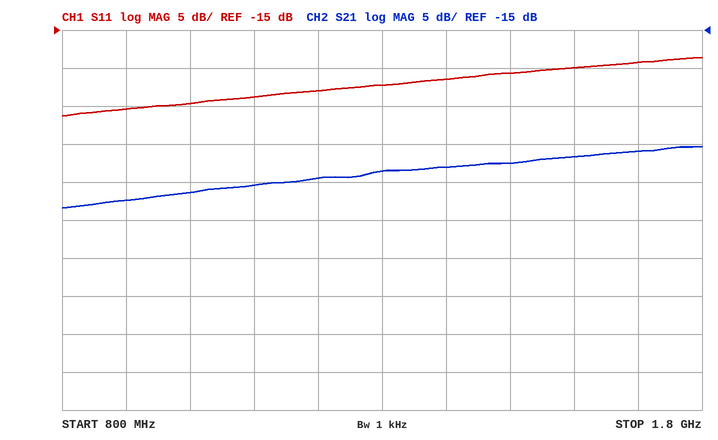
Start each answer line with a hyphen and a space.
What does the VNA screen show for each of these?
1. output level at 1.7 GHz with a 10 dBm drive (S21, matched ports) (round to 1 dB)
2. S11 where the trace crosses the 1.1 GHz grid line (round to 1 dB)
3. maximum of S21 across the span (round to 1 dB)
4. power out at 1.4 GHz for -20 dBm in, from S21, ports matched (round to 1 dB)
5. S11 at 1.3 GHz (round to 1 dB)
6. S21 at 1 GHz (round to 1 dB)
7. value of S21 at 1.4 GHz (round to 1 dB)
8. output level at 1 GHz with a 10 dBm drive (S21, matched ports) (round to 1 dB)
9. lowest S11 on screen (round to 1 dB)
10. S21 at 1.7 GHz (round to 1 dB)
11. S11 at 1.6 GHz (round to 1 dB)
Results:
- -21 dBm
- -24 dB
- -30 dB
- -53 dBm
- -22 dB
- -36 dB
- -33 dB
- -26 dBm
- -26 dB
- -31 dB
- -20 dB
